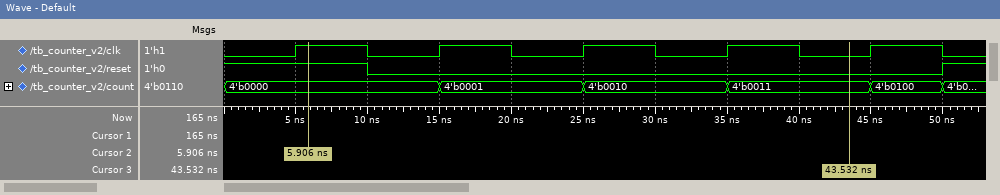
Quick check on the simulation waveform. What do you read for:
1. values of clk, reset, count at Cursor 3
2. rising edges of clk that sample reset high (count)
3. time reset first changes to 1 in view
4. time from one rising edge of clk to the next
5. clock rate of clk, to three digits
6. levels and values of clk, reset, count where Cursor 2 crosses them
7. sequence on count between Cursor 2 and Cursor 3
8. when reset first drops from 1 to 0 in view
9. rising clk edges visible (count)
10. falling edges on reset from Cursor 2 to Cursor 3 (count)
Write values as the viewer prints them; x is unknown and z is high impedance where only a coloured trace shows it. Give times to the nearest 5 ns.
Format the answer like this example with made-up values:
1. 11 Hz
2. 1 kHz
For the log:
1. clk=0, reset=0, count=4'b0011
2. 1
3. 50 ns
4. 10 ns
5. 100 MHz
6. clk=1, reset=1, count=4'b0000
7. 4'b0000, 4'b0001, 4'b0010, 4'b0011
8. 10 ns
9. 5
10. 1
